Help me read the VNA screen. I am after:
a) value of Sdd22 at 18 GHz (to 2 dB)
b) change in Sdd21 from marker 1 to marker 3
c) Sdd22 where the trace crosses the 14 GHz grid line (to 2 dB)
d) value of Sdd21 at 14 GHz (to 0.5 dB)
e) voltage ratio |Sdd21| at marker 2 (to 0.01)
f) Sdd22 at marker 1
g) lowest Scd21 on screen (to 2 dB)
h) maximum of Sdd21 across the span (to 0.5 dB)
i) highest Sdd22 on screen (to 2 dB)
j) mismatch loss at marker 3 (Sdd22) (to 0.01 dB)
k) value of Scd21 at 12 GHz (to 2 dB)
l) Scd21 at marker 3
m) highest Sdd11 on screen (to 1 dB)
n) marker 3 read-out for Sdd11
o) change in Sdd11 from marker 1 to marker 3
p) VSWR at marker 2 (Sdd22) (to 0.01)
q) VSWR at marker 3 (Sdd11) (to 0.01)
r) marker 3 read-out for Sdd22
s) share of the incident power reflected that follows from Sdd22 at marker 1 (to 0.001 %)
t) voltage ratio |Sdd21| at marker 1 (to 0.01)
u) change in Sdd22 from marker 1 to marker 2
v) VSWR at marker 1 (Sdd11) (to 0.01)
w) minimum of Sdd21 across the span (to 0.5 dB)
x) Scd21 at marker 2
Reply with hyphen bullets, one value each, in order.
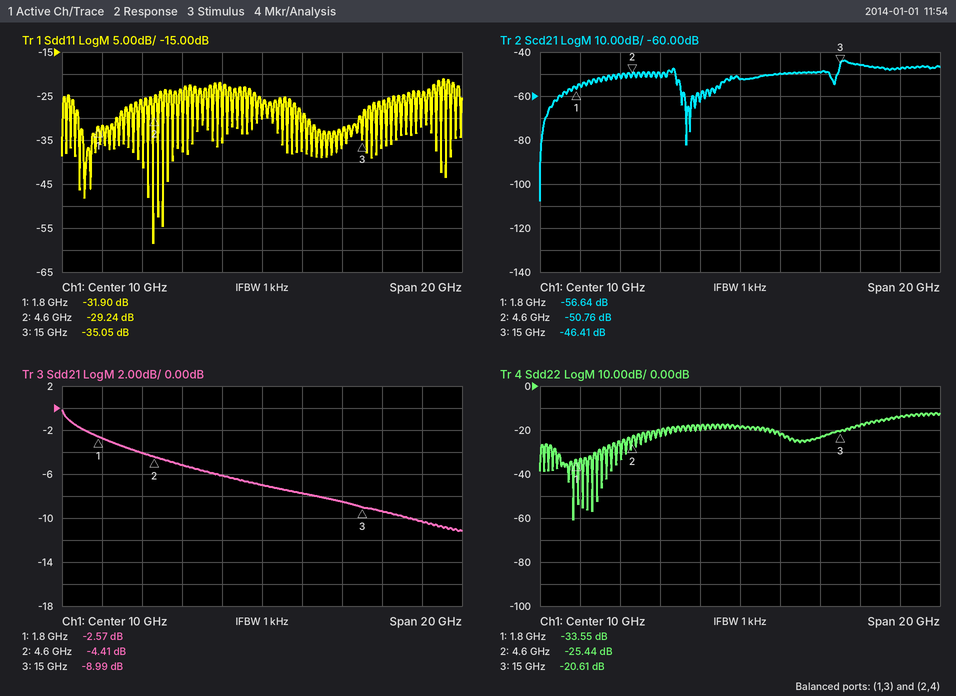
- -14 dB
- -6.42 dB
- -24 dB
- -8.5 dB
- 0.60
- -33.55 dB
- -108 dB
- 0.0 dB
- -12 dB
- 0.04 dB
- -50 dB
- -46.41 dB
- -21 dB
- -35.05 dB
- -3.15 dB
- 1.11
- 1.04
- -20.61 dB
- 0.044 %
- 0.74
- 8.11 dB
- 1.05
- -11.0 dB
- -50.76 dB
